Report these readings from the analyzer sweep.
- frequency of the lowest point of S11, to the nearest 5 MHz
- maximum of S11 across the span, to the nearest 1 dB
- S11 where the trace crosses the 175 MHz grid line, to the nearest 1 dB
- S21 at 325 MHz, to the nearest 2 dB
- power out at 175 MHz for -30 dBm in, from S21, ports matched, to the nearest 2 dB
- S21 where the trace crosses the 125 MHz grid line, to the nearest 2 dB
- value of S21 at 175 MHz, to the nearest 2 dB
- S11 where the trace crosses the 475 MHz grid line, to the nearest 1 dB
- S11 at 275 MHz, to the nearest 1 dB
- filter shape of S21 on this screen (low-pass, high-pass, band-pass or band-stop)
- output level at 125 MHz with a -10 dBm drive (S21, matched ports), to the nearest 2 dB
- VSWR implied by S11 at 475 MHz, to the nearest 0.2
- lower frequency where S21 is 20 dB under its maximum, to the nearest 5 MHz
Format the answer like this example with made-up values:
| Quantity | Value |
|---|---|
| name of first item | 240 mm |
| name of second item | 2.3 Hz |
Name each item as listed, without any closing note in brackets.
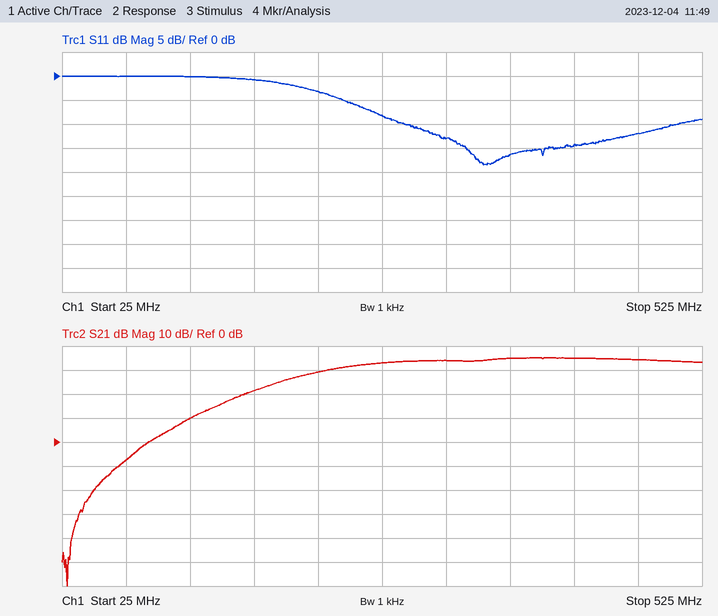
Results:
| Quantity | Value |
|---|---|
| frequency of the lowest point of S11, to the nearest 5 MHz | 355 MHz |
| maximum of S11 across the span, to the nearest 1 dB | 0 dB |
| S11 where the trace crosses the 175 MHz grid line, to the nearest 1 dB | -1 dB |
| S21 at 325 MHz, to the nearest 2 dB | 34 dB |
| power out at 175 MHz for -30 dBm in, from S21, ports matched, to the nearest 2 dB | -8 dBm |
| S21 where the trace crosses the 125 MHz grid line, to the nearest 2 dB | 10 dB |
| value of S21 at 175 MHz, to the nearest 2 dB | 22 dB |
| S11 where the trace crosses the 475 MHz grid line, to the nearest 1 dB | -12 dB |
| S11 at 275 MHz, to the nearest 1 dB | -8 dB |
| filter shape of S21 on this screen | high-pass |
| output level at 125 MHz with a -10 dBm drive (S21, matched ports), to the nearest 2 dB | 0 dBm |
| VSWR implied by S11 at 475 MHz, to the nearest 0.2 | 1.6 |
| lower frequency where S21 is 20 dB under its maximum, to the nearest 5 MHz | 145 MHz |
